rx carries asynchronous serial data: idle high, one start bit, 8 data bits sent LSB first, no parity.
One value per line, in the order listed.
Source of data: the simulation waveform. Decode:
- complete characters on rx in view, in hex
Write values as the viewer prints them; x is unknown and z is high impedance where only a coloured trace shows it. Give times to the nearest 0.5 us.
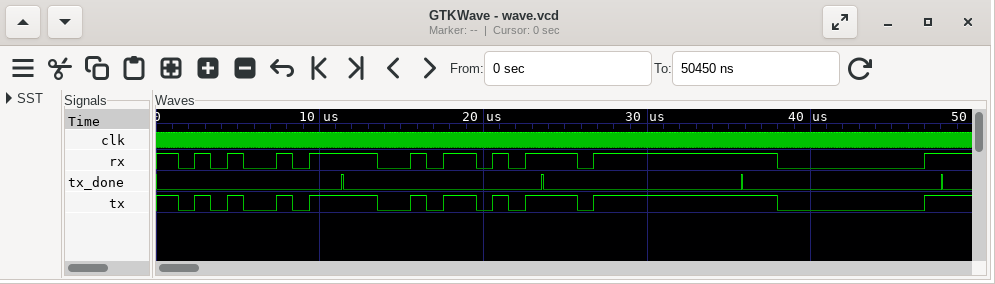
A5, 5A, FF, 00
